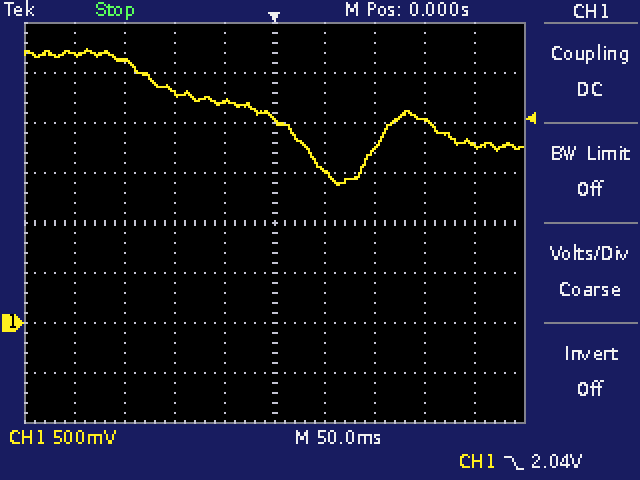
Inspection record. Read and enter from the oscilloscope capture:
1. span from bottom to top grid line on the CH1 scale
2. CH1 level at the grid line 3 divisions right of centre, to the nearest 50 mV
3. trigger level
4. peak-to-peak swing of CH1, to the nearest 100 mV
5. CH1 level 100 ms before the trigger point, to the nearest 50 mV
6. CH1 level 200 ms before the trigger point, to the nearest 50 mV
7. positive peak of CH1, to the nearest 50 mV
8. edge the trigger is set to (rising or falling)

4 V
2.05 V
2.04 V
1.40 V
2.30 V
2.70 V
2.75 V
falling
